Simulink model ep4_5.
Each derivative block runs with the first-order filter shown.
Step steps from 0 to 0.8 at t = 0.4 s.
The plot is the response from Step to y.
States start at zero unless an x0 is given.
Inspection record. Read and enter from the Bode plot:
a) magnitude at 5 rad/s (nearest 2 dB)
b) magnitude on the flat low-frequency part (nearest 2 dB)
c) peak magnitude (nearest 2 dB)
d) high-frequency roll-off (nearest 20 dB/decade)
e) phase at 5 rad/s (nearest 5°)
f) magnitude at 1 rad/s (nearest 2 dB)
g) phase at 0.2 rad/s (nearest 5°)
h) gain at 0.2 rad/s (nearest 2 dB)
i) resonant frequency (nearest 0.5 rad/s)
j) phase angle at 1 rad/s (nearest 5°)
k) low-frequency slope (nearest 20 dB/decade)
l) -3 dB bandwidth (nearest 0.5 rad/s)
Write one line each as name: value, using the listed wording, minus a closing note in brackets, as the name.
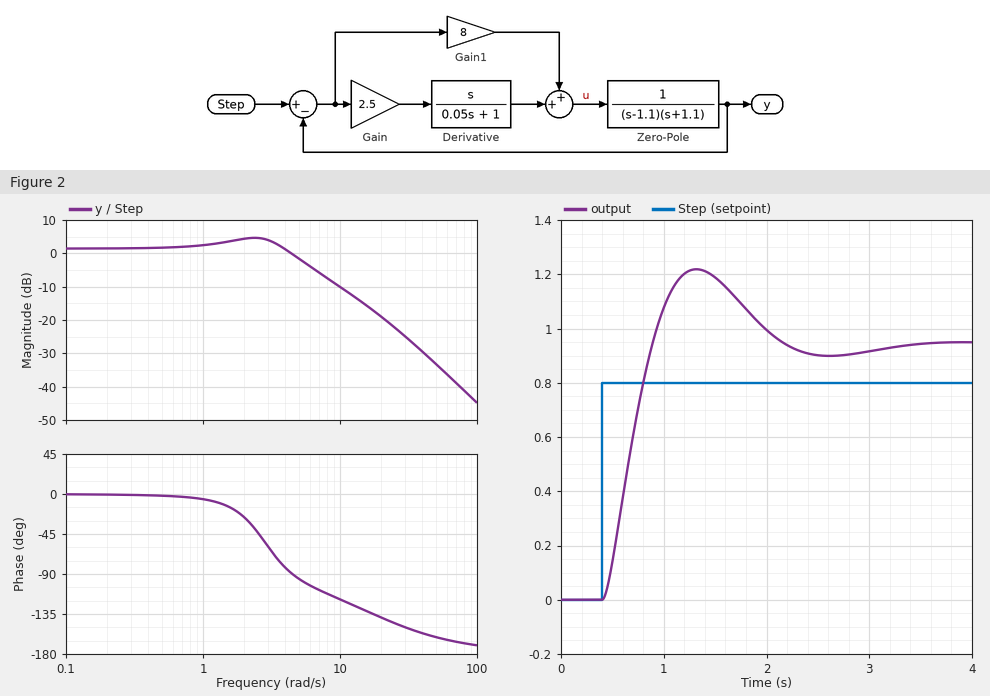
magnitude at 5 rad/s: -2 dB
magnitude on the flat low-frequency part: 2 dB
peak magnitude: 4 dB
high-frequency roll-off: -40 dB/decade
phase at 5 rad/s: -95°
magnitude at 1 rad/s: 2 dB
phase at 0.2 rad/s: 0°
gain at 0.2 rad/s: 2 dB
resonant frequency: 2.5 rad/s
phase angle at 1 rad/s: -5°
low-frequency slope: 0 dB/decade
-3 dB bandwidth: 5.0 rad/s
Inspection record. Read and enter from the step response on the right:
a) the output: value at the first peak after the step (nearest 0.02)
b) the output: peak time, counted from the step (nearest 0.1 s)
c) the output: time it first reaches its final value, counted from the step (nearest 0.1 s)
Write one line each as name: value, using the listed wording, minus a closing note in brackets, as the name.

the output: value at the first peak after the step: 1.22
the output: peak time, counted from the step: 0.9 s
the output: time it first reaches its final value, counted from the step: 0.5 s
